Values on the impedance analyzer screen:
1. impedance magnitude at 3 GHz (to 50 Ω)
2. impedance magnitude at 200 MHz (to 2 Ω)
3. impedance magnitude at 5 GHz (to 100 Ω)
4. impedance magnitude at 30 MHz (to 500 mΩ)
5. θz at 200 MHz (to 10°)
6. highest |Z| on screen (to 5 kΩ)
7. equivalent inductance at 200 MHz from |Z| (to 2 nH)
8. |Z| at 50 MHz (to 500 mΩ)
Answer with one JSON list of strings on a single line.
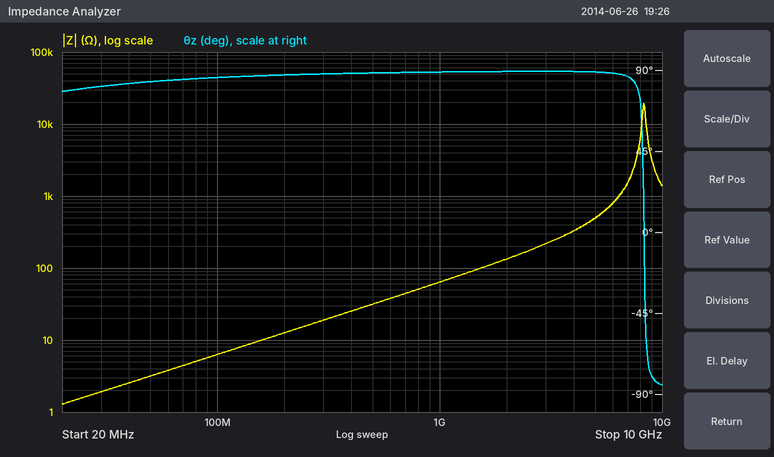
["200 Ω", "12 Ω", "500 Ω", "2.0 Ω", "90°", "20 kΩ", "10 nH", "3.0 Ω"]
